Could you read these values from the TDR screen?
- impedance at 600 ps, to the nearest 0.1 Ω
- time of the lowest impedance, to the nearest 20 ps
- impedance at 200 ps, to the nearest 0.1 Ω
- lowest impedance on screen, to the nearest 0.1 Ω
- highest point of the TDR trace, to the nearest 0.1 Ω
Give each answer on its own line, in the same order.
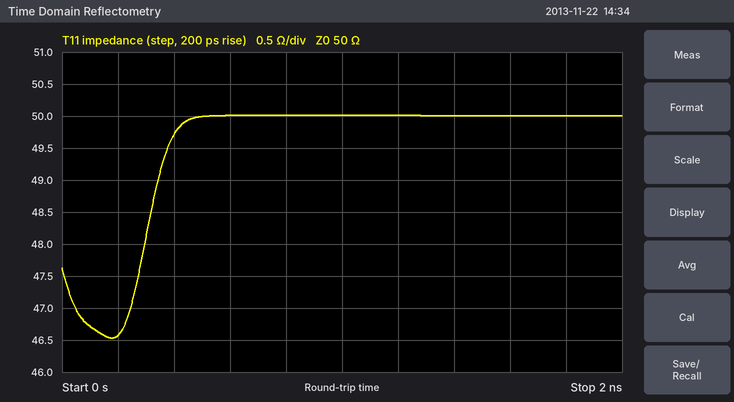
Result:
50.0 Ω
180 ps
46.6 Ω
46.5 Ω
50.0 Ω
